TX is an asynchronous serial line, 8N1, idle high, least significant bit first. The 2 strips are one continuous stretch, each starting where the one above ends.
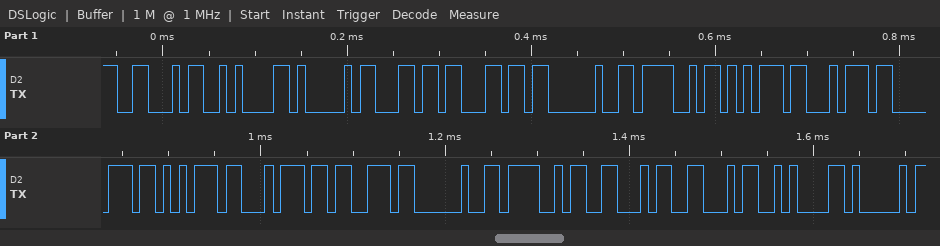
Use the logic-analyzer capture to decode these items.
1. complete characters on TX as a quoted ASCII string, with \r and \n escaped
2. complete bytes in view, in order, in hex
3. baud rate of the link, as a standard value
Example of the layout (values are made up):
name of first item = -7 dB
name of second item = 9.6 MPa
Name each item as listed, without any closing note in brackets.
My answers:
complete characters on TX as a quoted ASCII string, with \r and \n escaped = "F\nAll Outputs OFF\nA"
complete bytes in view, in order, in hex = 0x46 0x0A 0x41 0x6C 0x6C 0x20 0x4F 0x75 0x74 0x70 0x75 0x74 0x73 0x20 0x4F 0x46 0x46 0x0A 0x41
baud rate of the link, as a standard value = 115200 baud
